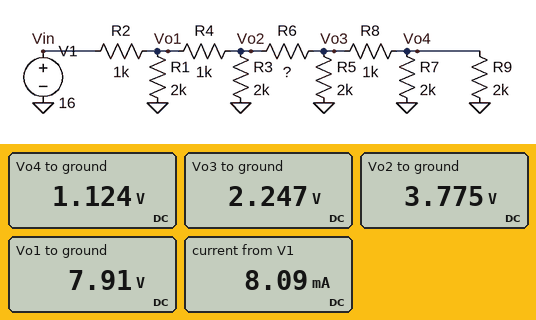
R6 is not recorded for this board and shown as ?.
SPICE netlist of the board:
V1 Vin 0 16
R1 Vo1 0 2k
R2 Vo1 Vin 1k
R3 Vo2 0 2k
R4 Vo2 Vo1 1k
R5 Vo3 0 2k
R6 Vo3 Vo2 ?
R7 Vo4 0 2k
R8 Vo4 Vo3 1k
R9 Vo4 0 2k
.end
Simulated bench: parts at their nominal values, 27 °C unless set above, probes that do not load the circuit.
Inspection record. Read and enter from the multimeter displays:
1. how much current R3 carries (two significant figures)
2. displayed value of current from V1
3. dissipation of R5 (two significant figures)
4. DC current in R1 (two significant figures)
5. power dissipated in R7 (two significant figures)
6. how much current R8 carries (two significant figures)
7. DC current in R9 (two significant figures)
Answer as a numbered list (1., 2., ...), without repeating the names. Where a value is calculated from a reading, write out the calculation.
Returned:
1. (3.775 V) / 2 kΩ = 1.9 mA
2. 8.09 mA
3. (2.247 V)^2 / 2 kΩ = 2.5 mW
4. (7.91 V) / 2 kΩ = 4.0 mA
5. (1.124 V)^2 / 2 kΩ = 630 µW
6. (2.247 V - 1.124 V) / 1 kΩ = 1.1 mA
7. (1.124 V) / 2 kΩ = 560 µA
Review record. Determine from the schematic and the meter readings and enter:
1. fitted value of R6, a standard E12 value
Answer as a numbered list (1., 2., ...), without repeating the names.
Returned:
1. 680 Ω
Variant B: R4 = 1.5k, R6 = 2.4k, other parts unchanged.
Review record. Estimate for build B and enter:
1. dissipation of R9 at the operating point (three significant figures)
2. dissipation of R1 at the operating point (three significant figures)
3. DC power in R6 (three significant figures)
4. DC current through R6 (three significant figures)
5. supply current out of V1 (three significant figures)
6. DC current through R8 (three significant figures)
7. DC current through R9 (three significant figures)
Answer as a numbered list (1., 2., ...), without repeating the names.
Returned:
1. 166 µW
2. 36.9 mW
3. 3.19 mW
4. 1.15 mA
5. 7.41 mA
6. 577 µA
7. 288 µA
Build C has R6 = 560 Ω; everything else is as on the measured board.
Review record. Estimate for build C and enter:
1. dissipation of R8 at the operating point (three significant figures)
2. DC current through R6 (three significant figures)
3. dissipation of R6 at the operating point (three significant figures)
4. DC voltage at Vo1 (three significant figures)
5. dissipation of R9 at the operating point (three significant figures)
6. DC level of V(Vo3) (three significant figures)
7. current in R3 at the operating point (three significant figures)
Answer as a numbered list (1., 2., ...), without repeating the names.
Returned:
1. 1.39 mW
2. 2.36 mA
3. 3.11 mW
4. 7.87 V
5. 694 µW
6. 2.36 V
7. 1.84 mA
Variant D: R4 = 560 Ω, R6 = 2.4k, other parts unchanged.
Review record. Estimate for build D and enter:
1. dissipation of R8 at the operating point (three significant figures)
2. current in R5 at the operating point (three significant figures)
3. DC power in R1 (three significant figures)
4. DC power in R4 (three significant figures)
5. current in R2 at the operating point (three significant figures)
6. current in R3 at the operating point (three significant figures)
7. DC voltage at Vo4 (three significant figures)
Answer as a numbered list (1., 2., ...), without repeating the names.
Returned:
1. 631 µW
2. 795 µA
3. 30.5 mW
4. 10.3 mW
5. 8.19 mA
6. 2.70 mA
7. 795 mV
